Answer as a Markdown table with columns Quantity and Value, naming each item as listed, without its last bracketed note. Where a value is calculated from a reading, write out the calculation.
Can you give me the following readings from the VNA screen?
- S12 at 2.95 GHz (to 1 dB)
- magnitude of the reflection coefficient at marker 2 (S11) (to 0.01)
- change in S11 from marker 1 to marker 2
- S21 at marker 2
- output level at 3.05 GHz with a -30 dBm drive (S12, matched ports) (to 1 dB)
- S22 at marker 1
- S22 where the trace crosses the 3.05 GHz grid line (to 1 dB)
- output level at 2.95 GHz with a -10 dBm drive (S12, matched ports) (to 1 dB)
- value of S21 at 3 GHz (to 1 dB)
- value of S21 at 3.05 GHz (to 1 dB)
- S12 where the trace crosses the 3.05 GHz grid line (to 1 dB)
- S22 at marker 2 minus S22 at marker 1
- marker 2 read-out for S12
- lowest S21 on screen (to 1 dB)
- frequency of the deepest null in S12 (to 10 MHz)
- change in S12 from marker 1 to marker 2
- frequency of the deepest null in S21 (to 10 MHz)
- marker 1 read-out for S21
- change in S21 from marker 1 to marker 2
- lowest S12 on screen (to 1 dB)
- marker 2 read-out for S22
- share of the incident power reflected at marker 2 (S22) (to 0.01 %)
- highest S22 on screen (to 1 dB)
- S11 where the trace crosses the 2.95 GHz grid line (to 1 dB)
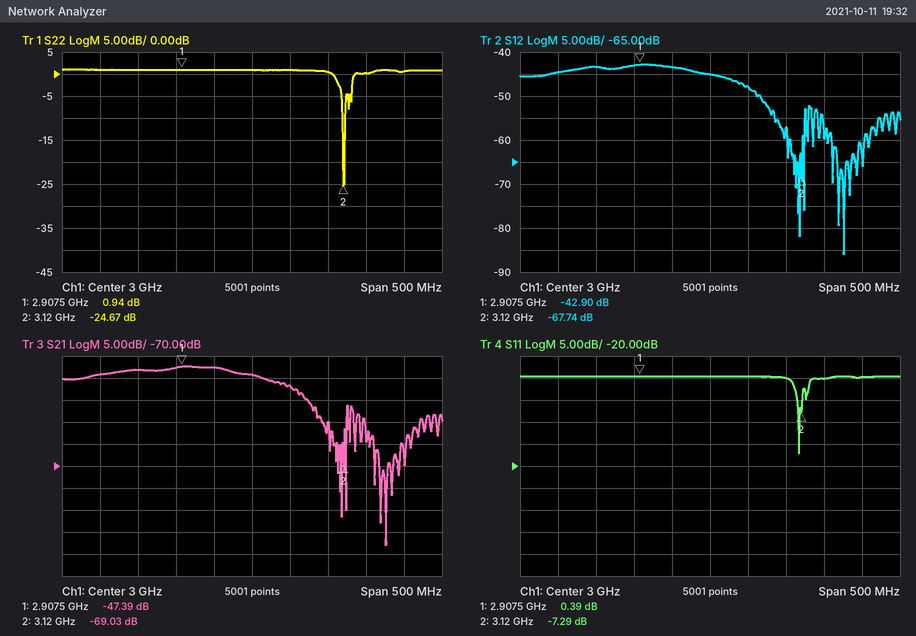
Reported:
| Quantity | Value |
|---|---|
| S12 at 2.95 GHz | -43 dB |
| magnitude of the reflection coefficient at marker 2 (S11) | 10^(-7.29/20) ≈ 0.43 |
| change in S11 from marker 1 to marker 2 | -7.29 − (0.39) = -7.68 dB |
| S21 at marker 2 | -69.03 dB |
| output level at 3.05 GHz with a -30 dBm drive (S12, matched ports) | -30 dBm + (-48 dB) = -78 dBm |
| S22 at marker 1 | 0.94 dB |
| S22 where the trace crosses the 3.05 GHz grid line | 1 dB |
| output level at 2.95 GHz with a -10 dBm drive (S12, matched ports) | -10 dBm + (-43 dB) = -53 dBm |
| value of S21 at 3 GHz | -49 dB |
| value of S21 at 3.05 GHz | -52 dB |
| S12 where the trace crosses the 3.05 GHz grid line | -48 dB |
| S22 at marker 2 minus S22 at marker 1 | -24.67 − (0.94) = -25.61 dB |
| marker 2 read-out for S12 | -67.74 dB |
| lowest S21 on screen | -88 dB |
| frequency of the deepest null in S12 | 3.18 GHz |
| change in S12 from marker 1 to marker 2 | -67.74 − (-42.9) = -24.84 dB |
| frequency of the deepest null in S21 | 3.18 GHz |
| marker 1 read-out for S21 | -47.39 dB |
| change in S21 from marker 1 to marker 2 | -69.03 − (-47.39) = -21.64 dB |
| lowest S12 on screen | -86 dB |
| marker 2 read-out for S22 | -24.67 dB |
| share of the incident power reflected at marker 2 (S22) | 10^(-24.67/10) ≈ 0.34 % |
| highest S22 on screen | 1 dB |
| S11 where the trace crosses the 2.95 GHz grid line | 0 dB |
